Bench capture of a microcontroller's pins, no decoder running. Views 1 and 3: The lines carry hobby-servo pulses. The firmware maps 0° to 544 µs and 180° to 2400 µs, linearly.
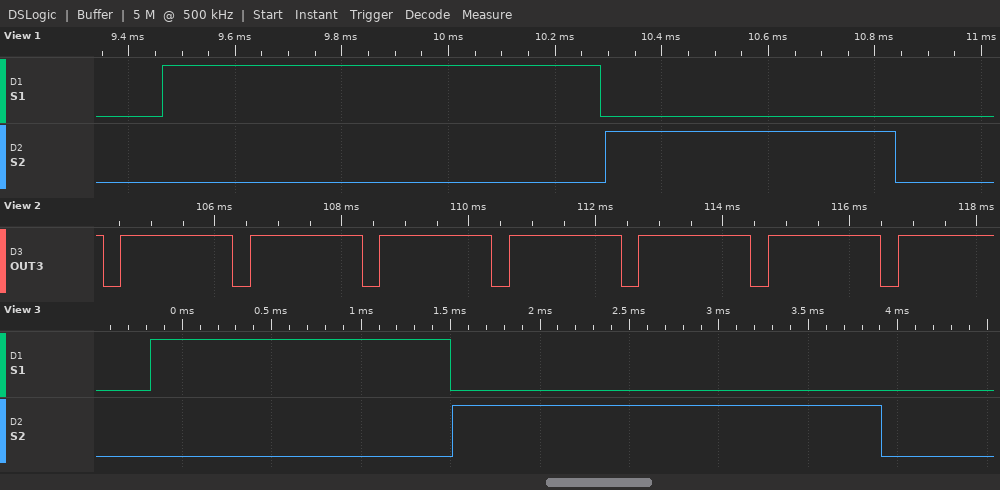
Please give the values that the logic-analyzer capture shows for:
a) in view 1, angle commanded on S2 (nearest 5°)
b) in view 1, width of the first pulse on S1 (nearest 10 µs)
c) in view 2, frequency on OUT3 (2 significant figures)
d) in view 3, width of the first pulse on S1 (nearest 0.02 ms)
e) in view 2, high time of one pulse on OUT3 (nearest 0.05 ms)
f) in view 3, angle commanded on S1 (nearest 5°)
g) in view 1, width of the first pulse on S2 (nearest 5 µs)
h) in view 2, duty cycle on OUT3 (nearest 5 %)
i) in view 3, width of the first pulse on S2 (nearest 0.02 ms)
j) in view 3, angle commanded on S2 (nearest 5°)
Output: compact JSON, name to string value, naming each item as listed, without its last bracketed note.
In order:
{"in view 1, angle commanded on S2": "0°", "in view 1, width of the first pulse on S1": "820 µs", "in view 2, frequency on OUT3": "490 Hz", "in view 3, width of the first pulse on S1": "1.68 ms", "in view 2, high time of one pulse on OUT3": "1.75 ms", "in view 3, angle commanded on S1": "110°", "in view 1, width of the first pulse on S2": "545 µs", "in view 2, duty cycle on OUT3": "85 %", "in view 3, width of the first pulse on S2": "2.40 ms", "in view 3, angle commanded on S2": "180°"}
